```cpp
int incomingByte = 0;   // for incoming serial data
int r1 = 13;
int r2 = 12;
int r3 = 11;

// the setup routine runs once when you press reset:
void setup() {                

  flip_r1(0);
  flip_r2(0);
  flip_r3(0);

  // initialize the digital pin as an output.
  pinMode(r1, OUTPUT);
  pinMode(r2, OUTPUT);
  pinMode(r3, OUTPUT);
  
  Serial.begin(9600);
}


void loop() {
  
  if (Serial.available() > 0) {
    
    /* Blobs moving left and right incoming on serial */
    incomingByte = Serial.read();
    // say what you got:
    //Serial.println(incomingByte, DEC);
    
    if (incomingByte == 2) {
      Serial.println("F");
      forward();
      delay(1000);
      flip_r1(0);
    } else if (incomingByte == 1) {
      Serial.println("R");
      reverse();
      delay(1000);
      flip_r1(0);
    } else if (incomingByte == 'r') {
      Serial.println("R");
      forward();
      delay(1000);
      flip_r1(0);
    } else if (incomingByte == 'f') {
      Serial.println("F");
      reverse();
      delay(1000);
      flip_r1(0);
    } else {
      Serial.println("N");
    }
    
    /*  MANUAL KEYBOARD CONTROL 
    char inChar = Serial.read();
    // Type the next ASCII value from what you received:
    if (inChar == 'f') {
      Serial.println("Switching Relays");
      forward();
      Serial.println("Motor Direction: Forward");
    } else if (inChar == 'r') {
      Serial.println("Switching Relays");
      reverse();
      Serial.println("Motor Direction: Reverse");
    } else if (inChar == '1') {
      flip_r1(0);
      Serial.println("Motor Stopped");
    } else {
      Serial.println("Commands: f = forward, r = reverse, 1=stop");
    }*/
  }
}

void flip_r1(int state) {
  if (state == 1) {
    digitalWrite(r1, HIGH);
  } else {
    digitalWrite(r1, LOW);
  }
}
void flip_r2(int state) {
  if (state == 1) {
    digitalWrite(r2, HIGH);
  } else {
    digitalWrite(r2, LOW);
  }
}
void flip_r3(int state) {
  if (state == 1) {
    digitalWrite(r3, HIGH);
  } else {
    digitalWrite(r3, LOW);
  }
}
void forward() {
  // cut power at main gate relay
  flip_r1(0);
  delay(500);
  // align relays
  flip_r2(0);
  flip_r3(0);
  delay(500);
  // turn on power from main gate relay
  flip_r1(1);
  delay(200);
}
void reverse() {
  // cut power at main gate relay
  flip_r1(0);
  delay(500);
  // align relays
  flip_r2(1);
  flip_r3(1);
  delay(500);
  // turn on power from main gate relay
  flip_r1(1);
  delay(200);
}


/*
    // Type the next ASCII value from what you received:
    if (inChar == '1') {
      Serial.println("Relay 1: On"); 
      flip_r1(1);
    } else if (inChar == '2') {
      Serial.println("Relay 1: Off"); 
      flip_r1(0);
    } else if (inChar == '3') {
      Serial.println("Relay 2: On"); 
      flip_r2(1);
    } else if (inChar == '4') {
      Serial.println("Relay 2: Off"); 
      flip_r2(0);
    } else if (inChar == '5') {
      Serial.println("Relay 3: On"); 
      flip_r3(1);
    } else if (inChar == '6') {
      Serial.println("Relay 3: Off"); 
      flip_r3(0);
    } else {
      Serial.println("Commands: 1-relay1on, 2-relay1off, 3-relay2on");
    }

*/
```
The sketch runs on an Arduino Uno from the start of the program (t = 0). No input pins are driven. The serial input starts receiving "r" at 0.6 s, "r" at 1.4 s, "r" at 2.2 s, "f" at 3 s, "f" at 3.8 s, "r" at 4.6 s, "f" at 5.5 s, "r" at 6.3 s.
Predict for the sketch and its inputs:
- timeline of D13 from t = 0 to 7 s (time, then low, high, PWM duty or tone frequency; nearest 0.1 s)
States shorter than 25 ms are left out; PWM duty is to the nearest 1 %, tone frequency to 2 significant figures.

0 s low; 1.6 s high; 2.8 s low; 3.8 s high; 5 s low; 6 s high
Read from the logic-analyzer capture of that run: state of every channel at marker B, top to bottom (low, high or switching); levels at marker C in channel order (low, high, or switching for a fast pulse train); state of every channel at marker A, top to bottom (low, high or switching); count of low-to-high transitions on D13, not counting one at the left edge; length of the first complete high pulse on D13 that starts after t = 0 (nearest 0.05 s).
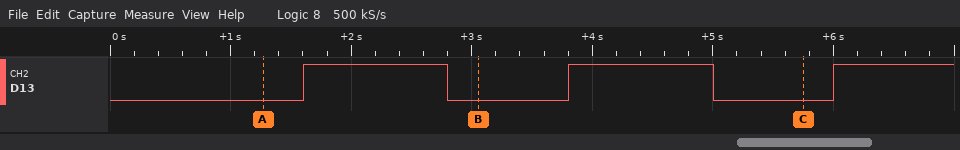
D13 low
D13 low
D13 low
3
1.20 s
